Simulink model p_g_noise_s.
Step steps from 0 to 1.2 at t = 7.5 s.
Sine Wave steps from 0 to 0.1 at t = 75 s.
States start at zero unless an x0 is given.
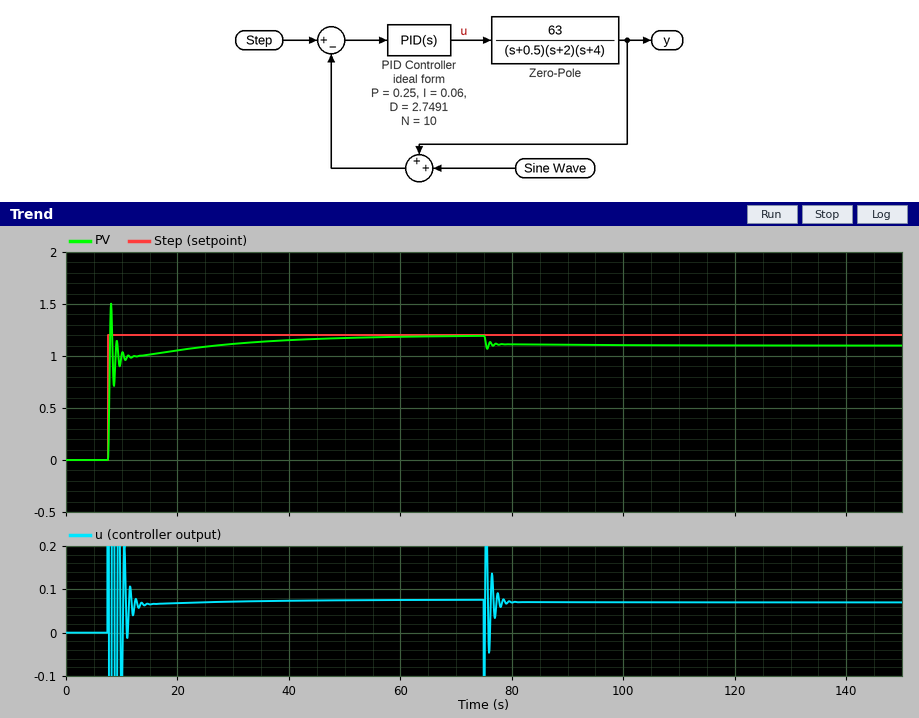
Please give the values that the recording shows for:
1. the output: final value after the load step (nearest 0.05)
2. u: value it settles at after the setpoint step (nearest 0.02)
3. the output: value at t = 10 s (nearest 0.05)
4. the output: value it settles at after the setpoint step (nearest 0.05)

1.10
0.08
1.00
1.20
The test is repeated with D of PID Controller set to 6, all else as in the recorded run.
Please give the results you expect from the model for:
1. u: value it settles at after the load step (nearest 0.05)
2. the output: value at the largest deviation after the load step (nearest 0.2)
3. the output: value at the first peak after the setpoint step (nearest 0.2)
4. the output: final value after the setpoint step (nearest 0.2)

0.05
1.0
2.0
1.2
